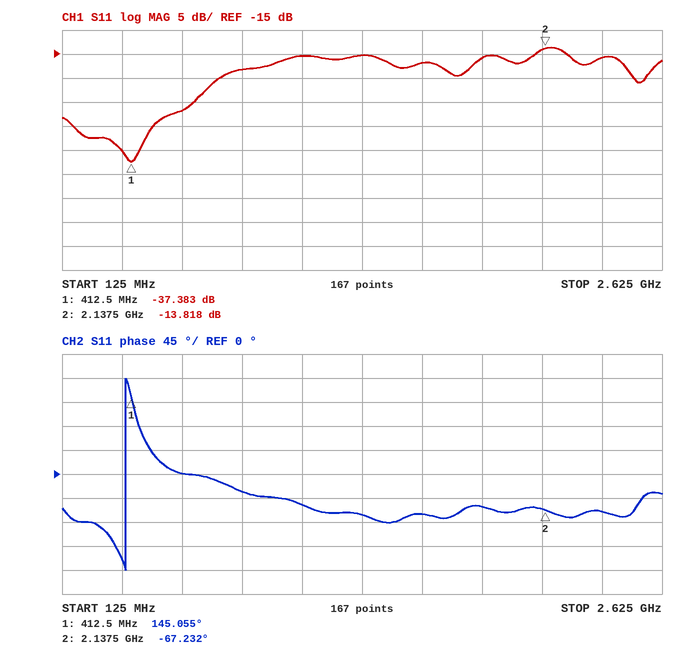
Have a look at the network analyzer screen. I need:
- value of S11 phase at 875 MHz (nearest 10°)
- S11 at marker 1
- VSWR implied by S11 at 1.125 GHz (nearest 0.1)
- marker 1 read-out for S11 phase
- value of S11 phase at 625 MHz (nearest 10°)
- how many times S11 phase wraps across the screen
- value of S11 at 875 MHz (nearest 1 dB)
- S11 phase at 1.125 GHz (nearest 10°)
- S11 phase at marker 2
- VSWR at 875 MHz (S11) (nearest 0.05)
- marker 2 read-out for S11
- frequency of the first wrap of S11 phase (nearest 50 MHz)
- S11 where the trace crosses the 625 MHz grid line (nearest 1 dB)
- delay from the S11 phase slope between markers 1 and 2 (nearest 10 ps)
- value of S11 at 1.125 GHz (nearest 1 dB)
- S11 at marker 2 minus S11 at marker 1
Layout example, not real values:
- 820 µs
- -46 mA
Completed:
- -30°
- -37.383 dB
- 1.4
- 145.055°
- 0°
- 1
- -18 dB
- -60°
- -67.232°
- 1.30
- -13.818 dB
- 400 MHz
- -27 dB
- 340 ps
- -15 dB
- 23.565 dB
